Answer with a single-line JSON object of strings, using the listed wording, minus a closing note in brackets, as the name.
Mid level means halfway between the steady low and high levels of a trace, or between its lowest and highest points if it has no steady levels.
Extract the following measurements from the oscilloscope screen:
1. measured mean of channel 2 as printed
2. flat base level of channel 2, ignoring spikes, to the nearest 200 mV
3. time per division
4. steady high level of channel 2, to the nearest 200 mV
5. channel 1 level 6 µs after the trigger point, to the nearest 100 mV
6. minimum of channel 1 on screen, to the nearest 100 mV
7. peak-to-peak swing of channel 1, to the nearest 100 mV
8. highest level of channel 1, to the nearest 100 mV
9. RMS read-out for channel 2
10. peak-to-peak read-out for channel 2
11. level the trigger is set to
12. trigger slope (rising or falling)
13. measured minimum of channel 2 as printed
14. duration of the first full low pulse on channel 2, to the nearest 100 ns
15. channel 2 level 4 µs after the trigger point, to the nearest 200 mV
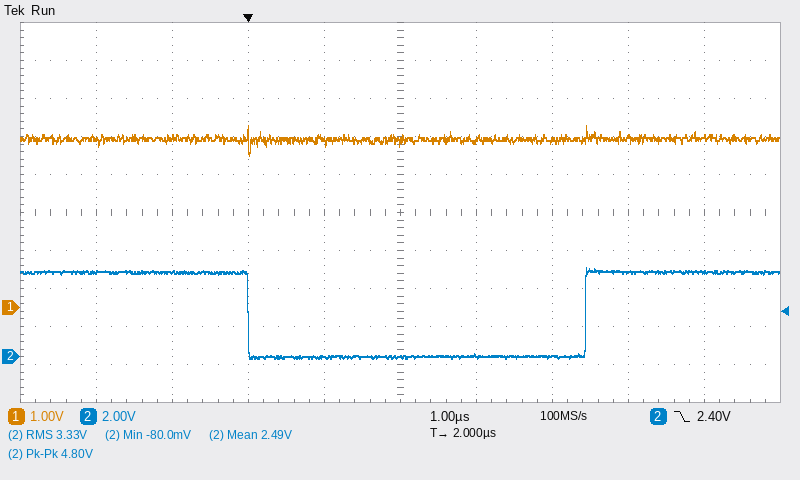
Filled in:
{"measured mean of channel 2 as printed": "2.49 V", "flat base level of channel 2, ignoring spikes, to the nearest 200 mV": "0.0 V", "time per division": "1 µs", "steady high level of channel 2, to the nearest 200 mV": "4.4 V", "channel 1 level 6 µs after the trigger point, to the nearest 100 mV": "4.5 V", "minimum of channel 1 on screen, to the nearest 100 mV": "4.0 V", "peak-to-peak swing of channel 1, to the nearest 100 mV": "800 mV", "highest level of channel 1, to the nearest 100 mV": "4.8 V", "RMS read-out for channel 2": "3.33 V", "peak-to-peak read-out for channel 2": "4.80 V", "level the trigger is set to": "2.40 V", "trigger slope": "falling", "measured minimum of channel 2 as printed": "-80.0 mV", "duration of the first full low pulse on channel 2, to the nearest 100 ns": "4.4 µs", "channel 2 level 4 µs after the trigger point, to the nearest 200 mV": "0.0 V"}
